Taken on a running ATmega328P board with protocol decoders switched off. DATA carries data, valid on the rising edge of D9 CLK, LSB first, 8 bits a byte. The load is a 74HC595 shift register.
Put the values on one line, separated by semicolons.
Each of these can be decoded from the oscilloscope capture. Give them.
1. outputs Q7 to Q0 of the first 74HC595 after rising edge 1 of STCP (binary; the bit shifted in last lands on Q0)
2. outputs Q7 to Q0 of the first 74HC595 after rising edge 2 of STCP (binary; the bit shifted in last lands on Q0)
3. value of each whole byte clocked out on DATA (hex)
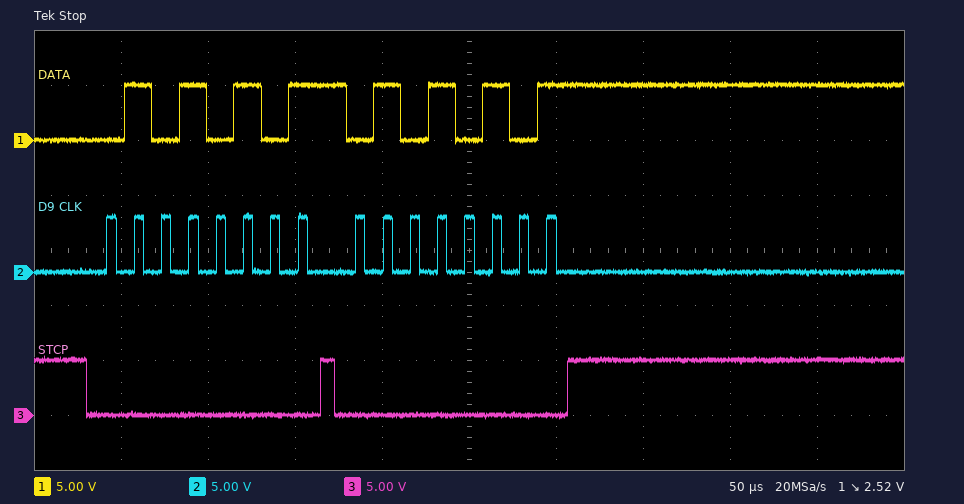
01010101; 01010101; 0xAA 0xAA
